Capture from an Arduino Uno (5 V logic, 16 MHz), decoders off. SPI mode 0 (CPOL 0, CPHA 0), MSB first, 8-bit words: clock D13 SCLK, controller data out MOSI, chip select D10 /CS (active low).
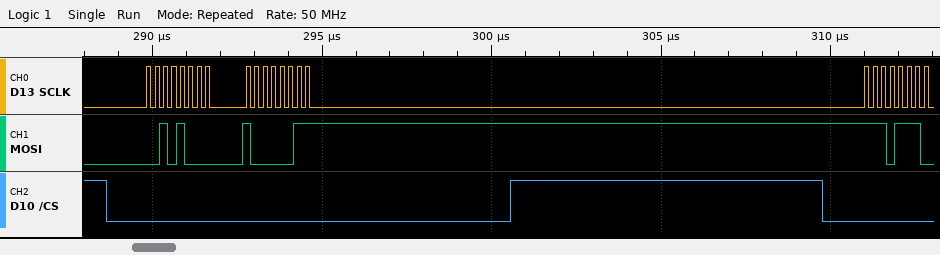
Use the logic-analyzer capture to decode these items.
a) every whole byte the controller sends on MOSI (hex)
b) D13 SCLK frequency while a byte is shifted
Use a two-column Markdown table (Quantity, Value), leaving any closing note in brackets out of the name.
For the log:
| Quantity | Value |
|---|---|
| every whole byte the controller sends on MOSI | 28 83 EE |
| D13 SCLK frequency while a byte is shifted | 4 MHz |
